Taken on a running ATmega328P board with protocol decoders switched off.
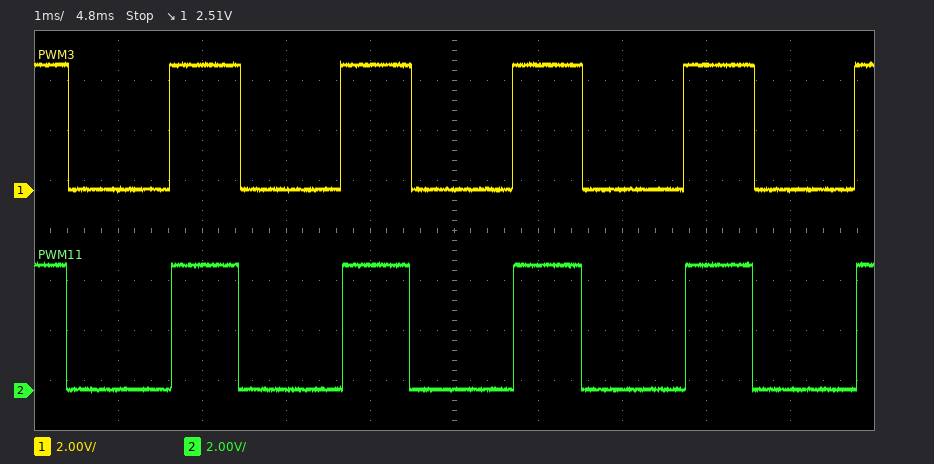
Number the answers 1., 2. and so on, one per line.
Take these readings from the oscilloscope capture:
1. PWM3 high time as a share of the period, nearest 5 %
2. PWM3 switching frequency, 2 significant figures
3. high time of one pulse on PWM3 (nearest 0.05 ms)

1. 40 %
2. 490 Hz
3. 0.85 ms
